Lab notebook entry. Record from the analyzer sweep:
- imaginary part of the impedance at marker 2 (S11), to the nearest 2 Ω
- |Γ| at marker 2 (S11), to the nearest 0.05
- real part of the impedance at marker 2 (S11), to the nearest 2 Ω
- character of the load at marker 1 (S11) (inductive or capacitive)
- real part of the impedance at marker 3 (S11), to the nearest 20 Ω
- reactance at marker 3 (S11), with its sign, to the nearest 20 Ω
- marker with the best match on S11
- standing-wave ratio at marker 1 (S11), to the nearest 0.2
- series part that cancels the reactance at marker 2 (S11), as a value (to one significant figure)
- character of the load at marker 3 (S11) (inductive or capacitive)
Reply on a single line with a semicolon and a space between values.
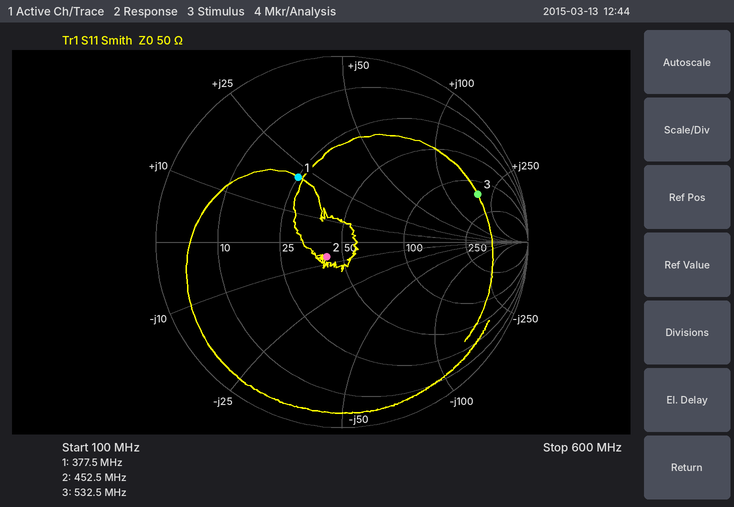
-6 Ω; 0.10; 42 Ω; inductive; 140 Ω; +180 Ω; marker 2; 2.4; 2 nH; inductive
